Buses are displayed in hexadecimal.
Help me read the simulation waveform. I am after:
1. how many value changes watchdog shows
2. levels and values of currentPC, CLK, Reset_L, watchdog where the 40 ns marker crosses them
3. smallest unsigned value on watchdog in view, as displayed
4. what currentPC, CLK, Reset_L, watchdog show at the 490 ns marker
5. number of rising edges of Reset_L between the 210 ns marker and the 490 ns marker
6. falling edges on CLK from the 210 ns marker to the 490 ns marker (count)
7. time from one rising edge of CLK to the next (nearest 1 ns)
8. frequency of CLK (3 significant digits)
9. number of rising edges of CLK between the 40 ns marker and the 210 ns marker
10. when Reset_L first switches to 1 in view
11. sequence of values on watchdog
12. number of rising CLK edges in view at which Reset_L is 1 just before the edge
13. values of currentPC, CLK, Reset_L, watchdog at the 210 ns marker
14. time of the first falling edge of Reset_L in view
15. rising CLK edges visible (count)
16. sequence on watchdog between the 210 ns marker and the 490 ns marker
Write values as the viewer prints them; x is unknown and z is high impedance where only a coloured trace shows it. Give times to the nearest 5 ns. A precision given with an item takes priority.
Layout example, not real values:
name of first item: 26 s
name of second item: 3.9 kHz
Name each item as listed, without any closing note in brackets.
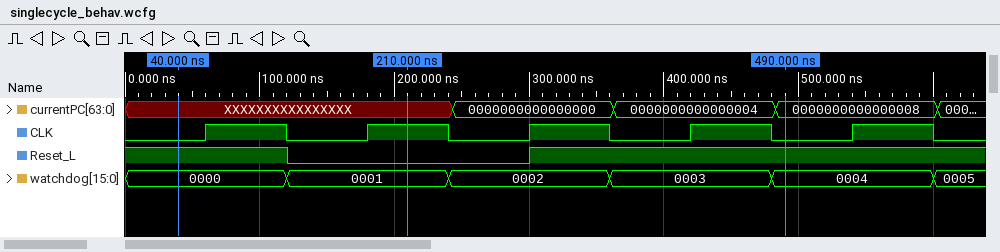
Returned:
how many value changes watchdog shows: 5
levels and values of currentPC, CLK, Reset_L, watchdog where the 40 ns marker crosses them: currentPC=XXXXXXXXXXXXXXXX, CLK=0, Reset_L=1, watchdog=0000
smallest unsigned value on watchdog in view, as displayed: 0000
what currentPC, CLK, Reset_L, watchdog show at the 490 ns marker: currentPC=0000000000000008, CLK=0, Reset_L=1, watchdog=0004
number of rising edges of Reset_L between the 210 ns marker and the 490 ns marker: 1
falling edges on CLK from the 210 ns marker to the 490 ns marker: 3
time from one rising edge of CLK to the next: 120 ns
frequency of CLK: 8.33 MHz
number of rising edges of CLK between the 40 ns marker and the 210 ns marker: 2
when Reset_L first switches to 1 in view: 300 ns
sequence of values on watchdog: 0000, 0001, 0002, 0003, 0004, 0005
number of rising CLK edges in view at which Reset_L is 1 just before the edge: 3
values of currentPC, CLK, Reset_L, watchdog at the 210 ns marker: currentPC=XXXXXXXXXXXXXXXX, CLK=1, Reset_L=0, watchdog=0001
time of the first falling edge of Reset_L in view: 120 ns
rising CLK edges visible: 5
sequence on watchdog between the 210 ns marker and the 490 ns marker: 0001, 0002, 0003, 0004
